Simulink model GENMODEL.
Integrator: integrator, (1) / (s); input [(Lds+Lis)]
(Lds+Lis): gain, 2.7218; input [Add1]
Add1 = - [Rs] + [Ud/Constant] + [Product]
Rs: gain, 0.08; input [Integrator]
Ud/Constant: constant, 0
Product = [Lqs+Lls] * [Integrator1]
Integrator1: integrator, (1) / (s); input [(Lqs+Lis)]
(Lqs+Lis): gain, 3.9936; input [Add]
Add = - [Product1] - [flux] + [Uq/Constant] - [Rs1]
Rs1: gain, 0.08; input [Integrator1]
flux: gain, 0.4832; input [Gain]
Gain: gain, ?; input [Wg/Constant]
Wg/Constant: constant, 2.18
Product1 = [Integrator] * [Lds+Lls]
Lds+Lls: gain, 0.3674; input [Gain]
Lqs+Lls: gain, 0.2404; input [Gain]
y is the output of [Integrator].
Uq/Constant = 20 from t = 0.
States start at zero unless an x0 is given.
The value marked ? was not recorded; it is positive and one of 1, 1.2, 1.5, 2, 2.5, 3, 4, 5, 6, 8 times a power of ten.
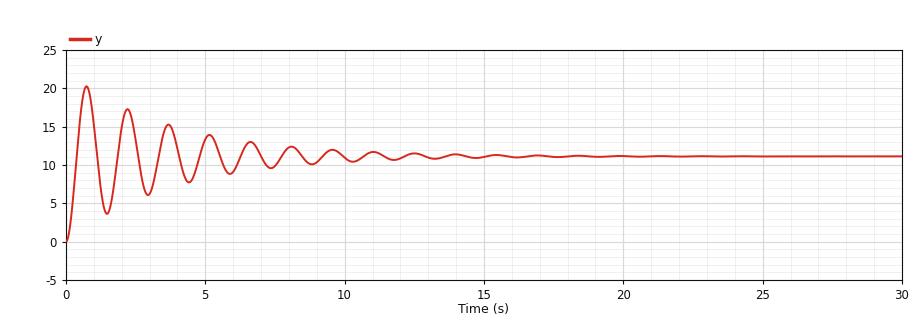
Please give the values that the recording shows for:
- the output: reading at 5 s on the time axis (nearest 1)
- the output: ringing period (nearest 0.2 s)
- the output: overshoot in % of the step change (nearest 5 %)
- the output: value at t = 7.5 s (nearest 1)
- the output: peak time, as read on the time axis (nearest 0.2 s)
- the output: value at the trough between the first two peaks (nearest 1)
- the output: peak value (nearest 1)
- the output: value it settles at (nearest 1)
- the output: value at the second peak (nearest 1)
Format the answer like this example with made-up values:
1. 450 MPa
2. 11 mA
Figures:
1. 13
2. 1.4 s
3. 80 %
4. 10
5. 0.8 s
6. 4
7. 20
8. 11
9. 17
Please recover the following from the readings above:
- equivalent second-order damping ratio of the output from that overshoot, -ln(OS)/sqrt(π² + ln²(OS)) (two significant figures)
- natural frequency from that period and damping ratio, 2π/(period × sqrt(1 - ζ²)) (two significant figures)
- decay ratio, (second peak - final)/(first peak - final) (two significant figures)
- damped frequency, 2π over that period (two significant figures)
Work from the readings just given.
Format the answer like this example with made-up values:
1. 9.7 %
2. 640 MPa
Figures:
1. 0.071
2. 4.5 rad/s
3. 0.67
4. 4.5 rad/s
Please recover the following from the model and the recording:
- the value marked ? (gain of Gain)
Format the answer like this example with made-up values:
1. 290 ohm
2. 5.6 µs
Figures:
1. 2
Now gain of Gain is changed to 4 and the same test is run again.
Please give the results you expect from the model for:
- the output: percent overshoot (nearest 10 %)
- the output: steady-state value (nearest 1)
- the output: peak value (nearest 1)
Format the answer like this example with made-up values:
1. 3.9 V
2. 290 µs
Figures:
1. 90 %
2. 5
3. 9
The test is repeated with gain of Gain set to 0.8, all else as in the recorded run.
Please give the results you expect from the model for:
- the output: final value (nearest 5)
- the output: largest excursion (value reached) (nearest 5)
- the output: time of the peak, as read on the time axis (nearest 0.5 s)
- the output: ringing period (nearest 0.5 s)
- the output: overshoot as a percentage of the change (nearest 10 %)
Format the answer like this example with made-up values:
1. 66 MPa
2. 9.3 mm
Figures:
1. 30
2. 45
3. 2.0 s
4. 3.5 s
5. 60 %
